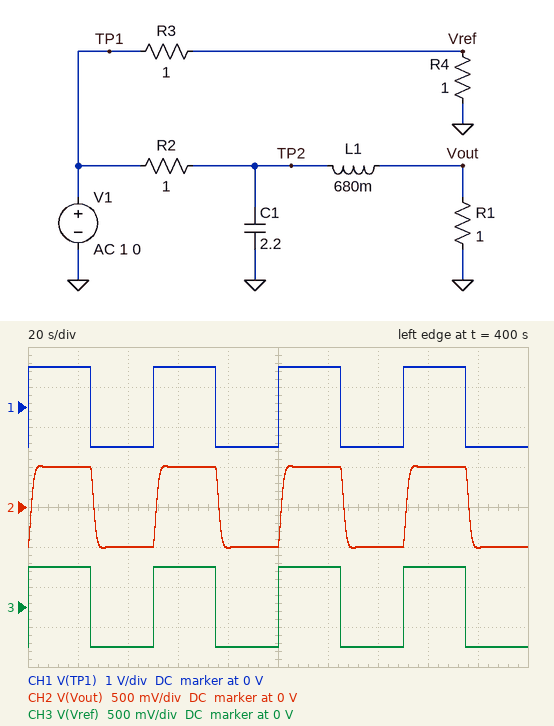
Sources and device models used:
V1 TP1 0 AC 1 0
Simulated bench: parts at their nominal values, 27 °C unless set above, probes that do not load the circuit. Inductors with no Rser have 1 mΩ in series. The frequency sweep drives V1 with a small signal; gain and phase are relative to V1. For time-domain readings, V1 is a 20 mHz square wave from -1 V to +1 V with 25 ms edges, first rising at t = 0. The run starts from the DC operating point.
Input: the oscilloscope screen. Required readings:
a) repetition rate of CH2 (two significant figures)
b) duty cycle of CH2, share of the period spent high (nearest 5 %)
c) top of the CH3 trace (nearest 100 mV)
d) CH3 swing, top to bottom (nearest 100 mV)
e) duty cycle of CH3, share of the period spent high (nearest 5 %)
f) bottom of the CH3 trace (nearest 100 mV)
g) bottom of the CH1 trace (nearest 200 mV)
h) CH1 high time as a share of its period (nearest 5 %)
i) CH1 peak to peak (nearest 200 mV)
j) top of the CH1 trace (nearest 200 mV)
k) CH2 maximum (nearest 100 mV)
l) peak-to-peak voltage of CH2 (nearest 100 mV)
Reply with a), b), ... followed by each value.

a) 20 mHz
b) 50 %
c) 500 mV
d) 1.0 V
e) 50 %
f) -500 mV
g) -1.0 V
h) 50 %
i) 2.0 V
j) 1.0 V
k) 500 mV
l) 1.0 V
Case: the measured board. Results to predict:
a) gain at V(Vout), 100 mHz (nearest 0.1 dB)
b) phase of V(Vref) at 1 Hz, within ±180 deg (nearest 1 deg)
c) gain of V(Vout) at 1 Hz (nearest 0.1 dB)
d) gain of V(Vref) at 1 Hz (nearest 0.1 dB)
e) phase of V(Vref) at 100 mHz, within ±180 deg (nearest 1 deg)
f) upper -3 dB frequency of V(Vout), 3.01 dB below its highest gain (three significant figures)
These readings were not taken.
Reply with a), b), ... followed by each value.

a) -7.2 dB
b) 0 deg
c) -35.5 dB
d) -6.0 dB
e) 0 deg
f) 152 mHz
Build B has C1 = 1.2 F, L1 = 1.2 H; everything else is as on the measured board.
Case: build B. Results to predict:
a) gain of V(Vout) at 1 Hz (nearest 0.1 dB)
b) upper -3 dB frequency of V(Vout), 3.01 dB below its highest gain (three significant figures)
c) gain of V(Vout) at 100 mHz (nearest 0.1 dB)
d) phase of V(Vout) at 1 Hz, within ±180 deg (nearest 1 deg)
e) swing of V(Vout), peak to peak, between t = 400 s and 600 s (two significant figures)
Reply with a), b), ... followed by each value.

a) -35.1 dB
b) 188 mHz
c) -6.4 dB
d) -165 deg
e) 1.1 V
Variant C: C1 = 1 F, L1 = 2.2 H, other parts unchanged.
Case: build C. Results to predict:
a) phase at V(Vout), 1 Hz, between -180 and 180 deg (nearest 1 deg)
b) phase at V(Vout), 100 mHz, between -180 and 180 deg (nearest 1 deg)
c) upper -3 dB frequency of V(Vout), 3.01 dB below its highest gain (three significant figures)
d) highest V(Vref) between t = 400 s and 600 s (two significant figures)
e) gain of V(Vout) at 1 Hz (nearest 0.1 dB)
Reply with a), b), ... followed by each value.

a) -167 deg
b) -61 deg
c) 140 mHz
d) 500 mV
e) -38.8 dB
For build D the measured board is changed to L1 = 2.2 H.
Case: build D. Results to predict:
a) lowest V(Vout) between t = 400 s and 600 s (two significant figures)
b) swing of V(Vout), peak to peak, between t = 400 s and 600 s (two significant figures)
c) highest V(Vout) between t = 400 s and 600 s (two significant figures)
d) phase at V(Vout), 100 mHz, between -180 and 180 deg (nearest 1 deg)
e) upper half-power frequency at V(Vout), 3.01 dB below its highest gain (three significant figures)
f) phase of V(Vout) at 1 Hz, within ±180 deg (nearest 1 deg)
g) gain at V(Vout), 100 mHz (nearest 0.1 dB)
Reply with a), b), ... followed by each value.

a) -540 mV
b) 1.1 V
c) 540 mV
d) -88 deg
e) 102 mHz
f) -172 deg
g) -8.8 dB
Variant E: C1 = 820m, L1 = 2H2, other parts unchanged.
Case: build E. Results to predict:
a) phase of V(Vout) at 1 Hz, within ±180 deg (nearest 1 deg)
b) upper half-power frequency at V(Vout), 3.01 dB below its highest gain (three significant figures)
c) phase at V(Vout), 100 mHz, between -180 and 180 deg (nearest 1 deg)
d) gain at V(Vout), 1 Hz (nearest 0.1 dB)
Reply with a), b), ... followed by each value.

a) -165 deg
b) 147 mHz
c) -56 deg
d) -37.1 dB
